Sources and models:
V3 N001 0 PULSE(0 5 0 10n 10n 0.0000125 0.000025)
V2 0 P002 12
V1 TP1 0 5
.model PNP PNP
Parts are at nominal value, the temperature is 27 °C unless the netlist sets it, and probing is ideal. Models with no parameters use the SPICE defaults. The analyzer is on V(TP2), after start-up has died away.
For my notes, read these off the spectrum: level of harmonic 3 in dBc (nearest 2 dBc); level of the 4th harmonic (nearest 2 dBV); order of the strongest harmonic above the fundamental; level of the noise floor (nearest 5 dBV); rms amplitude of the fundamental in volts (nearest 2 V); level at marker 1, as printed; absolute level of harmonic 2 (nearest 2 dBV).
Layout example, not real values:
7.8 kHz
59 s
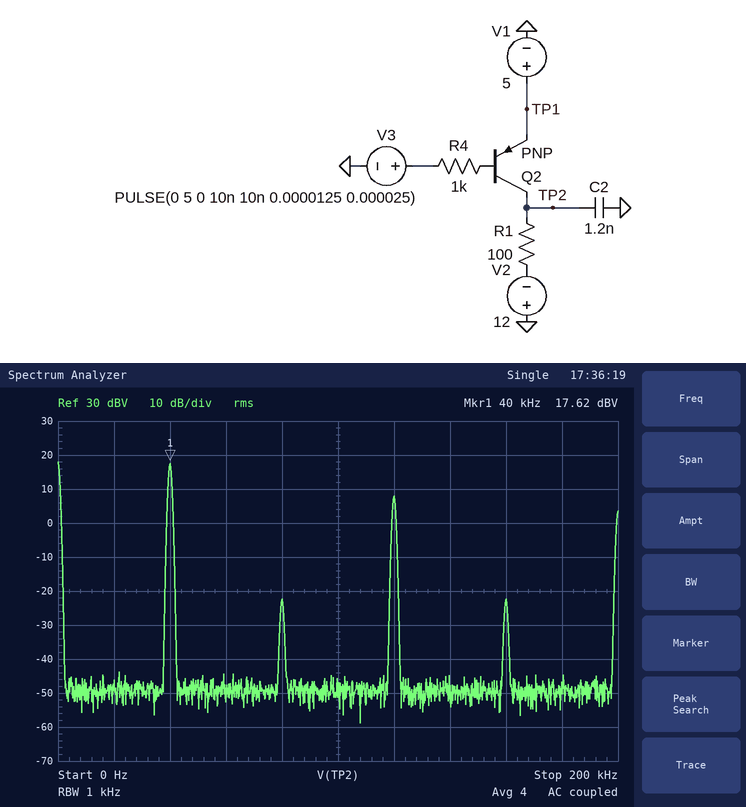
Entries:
-10 dBc
-22 dBV
3
-50 dBV
8 V
17.62 dBV
-22 dBV
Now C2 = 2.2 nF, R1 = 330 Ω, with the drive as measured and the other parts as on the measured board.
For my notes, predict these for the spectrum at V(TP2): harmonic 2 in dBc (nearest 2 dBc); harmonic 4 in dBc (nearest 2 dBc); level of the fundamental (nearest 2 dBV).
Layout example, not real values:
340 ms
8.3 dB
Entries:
-22 dBc
-24 dBc
18 dBV
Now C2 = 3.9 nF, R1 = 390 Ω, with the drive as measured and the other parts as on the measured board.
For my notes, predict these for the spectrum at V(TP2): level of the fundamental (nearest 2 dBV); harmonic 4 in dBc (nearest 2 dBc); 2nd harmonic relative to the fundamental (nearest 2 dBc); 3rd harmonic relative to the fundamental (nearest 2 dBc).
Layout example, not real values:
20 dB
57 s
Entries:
18 dBV
-20 dBc
-16 dBc
-12 dBc
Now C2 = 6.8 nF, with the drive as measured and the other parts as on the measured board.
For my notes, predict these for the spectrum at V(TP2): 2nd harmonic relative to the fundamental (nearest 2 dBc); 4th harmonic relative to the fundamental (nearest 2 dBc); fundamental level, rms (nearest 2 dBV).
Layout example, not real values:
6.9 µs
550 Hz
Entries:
-24 dBc
-26 dBc
18 dBV
